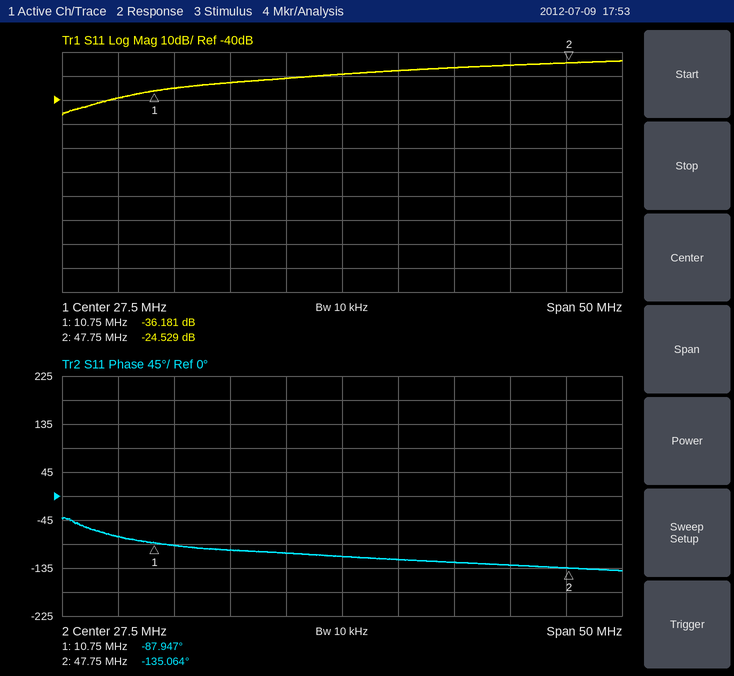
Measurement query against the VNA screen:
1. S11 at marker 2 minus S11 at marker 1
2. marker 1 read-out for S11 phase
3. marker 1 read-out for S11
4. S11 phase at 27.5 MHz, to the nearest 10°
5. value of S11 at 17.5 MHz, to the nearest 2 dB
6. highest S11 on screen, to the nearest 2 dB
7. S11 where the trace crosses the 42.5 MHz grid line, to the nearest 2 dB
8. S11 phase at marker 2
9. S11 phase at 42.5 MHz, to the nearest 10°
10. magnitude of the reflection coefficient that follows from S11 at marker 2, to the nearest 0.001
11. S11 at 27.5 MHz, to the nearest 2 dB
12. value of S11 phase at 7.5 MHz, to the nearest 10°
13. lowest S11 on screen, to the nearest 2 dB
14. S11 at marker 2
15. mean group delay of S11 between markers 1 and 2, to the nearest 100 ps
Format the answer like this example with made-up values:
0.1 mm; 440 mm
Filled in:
11.652 dB; -87.947°; -36.181 dB; -110°; -32 dB; -24 dB; -26 dB; -135.064°; -130°; 0.059; -30 dB; -80°; -46 dB; -24.529 dB; 3.5 ns
